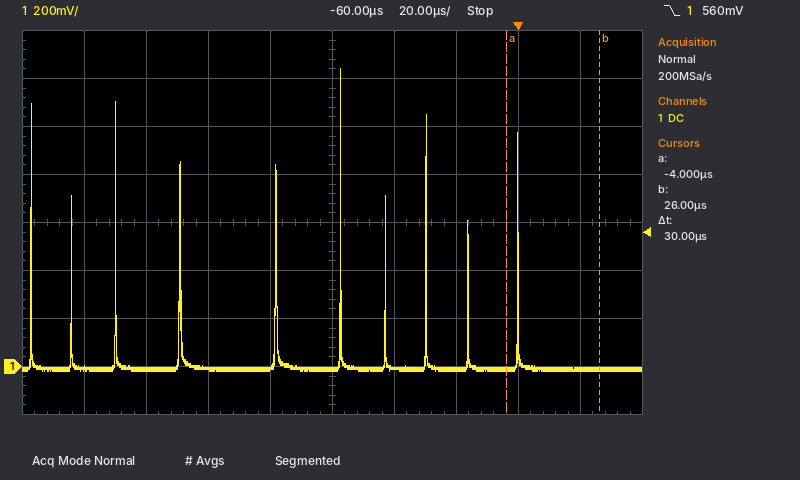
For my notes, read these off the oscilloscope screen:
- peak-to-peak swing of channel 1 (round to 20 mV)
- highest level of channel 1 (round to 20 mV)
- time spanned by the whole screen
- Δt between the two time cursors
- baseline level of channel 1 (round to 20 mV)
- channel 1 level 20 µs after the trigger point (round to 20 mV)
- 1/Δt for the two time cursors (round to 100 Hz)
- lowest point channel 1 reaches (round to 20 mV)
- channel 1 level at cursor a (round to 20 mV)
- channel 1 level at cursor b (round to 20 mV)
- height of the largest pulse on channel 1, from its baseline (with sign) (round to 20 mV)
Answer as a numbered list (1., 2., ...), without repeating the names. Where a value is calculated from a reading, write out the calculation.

1. 1.24 V − (-20 mV) = 1.26 V
2. 1.24 V
3. 200 µs
4. 30 µs
5. -20 mV
6. -20 mV
7. 1 / 30 µs ≈ 33.3 kHz
8. -20 mV
9. -20 mV
10. -20 mV
11. 1.24 V − (-20 mV) = +1.26 V
